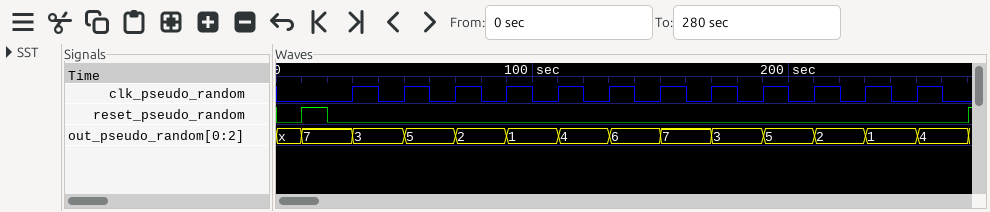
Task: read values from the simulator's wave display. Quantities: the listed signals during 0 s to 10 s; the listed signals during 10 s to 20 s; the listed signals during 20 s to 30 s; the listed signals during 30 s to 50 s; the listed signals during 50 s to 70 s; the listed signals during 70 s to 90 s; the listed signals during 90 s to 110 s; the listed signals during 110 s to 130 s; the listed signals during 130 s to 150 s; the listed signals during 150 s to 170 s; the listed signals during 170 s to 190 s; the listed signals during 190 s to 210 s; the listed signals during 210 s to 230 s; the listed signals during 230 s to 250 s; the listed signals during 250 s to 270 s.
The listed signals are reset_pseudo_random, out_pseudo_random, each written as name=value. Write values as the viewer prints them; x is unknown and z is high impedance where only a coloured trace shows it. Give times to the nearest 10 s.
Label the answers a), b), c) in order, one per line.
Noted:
a) reset_pseudo_random=0, out_pseudo_random=x
b) reset_pseudo_random=1, out_pseudo_random=7
c) reset_pseudo_random=0, out_pseudo_random=7
d) reset_pseudo_random=0, out_pseudo_random=3
e) reset_pseudo_random=0, out_pseudo_random=5
f) reset_pseudo_random=0, out_pseudo_random=2
g) reset_pseudo_random=0, out_pseudo_random=1
h) reset_pseudo_random=0, out_pseudo_random=4
i) reset_pseudo_random=0, out_pseudo_random=6
j) reset_pseudo_random=0, out_pseudo_random=7
k) reset_pseudo_random=0, out_pseudo_random=3
l) reset_pseudo_random=0, out_pseudo_random=5
m) reset_pseudo_random=0, out_pseudo_random=2
n) reset_pseudo_random=0, out_pseudo_random=1
o) reset_pseudo_random=0, out_pseudo_random=4
